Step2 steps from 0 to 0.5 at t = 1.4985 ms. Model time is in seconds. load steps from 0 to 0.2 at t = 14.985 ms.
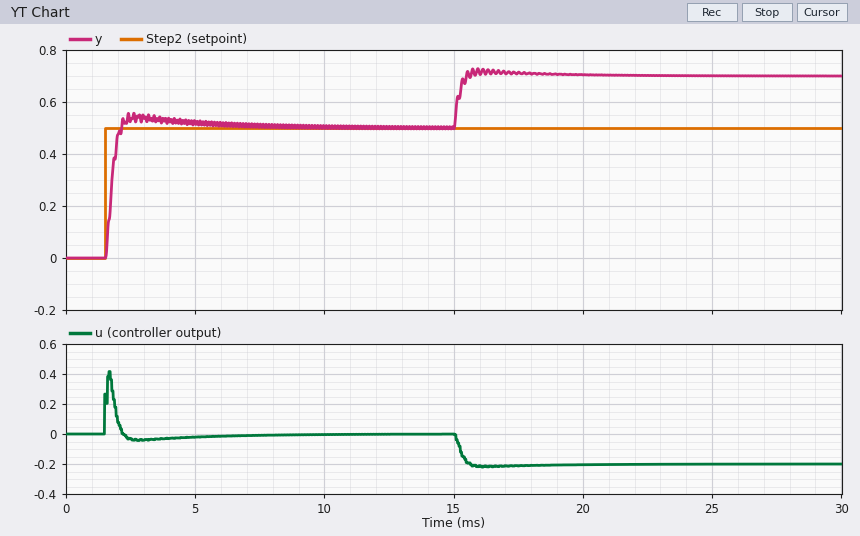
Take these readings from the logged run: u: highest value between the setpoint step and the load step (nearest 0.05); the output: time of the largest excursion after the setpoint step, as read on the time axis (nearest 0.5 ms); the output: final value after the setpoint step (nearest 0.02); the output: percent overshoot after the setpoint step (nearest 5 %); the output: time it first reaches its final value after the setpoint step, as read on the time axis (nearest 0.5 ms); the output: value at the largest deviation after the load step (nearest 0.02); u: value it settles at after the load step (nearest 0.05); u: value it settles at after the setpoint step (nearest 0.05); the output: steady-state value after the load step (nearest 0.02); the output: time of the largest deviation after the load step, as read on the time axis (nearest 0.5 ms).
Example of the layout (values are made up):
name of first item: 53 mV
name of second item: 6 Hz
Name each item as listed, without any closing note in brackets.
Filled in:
u: highest value between the setpoint step and the load step: 0.40
the output: time of the largest excursion after the setpoint step, as read on the time axis: 2.5 ms
the output: final value after the setpoint step: 0.50
the output: percent overshoot after the setpoint step: 10 %
the output: time it first reaches its final value after the setpoint step, as read on the time axis: 2.0 ms
the output: value at the largest deviation after the load step: 0.72
u: value it settles at after the load step: -0.20
u: value it settles at after the setpoint step: 0.00
the output: steady-state value after the load step: 0.70
the output: time of the largest deviation after the load step, as read on the time axis: 16.0 ms
